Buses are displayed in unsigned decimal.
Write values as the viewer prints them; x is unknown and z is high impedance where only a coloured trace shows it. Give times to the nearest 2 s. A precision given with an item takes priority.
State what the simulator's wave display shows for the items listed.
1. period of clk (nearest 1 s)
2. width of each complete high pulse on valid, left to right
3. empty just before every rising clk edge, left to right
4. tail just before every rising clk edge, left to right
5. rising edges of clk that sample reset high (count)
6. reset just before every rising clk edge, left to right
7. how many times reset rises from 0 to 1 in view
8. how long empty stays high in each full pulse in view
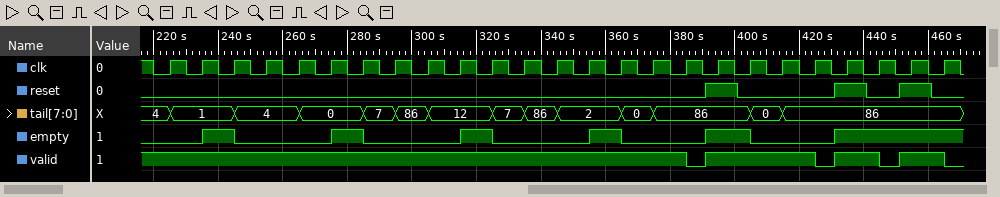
10 s
34 s, 14 s, 14 s
0 0 1 0 0 0 1 0 0 0 1 0 0 0 1 0 0 1 1 0 0 1 1 1 1
4, 1, 1, 4, 4, 0, 0, 7, 86, 12, 12, 7, 86, 2, 2, 0, 86, 86, 86, 0, 86, 86, 86, 86, 86
3
0 0 0 0 0 0 0 0 0 0 0 0 0 0 0 0 0 1 0 0 0 1 0 1 0
3
10 s, 10 s, 10 s, 10 s, 14 s
